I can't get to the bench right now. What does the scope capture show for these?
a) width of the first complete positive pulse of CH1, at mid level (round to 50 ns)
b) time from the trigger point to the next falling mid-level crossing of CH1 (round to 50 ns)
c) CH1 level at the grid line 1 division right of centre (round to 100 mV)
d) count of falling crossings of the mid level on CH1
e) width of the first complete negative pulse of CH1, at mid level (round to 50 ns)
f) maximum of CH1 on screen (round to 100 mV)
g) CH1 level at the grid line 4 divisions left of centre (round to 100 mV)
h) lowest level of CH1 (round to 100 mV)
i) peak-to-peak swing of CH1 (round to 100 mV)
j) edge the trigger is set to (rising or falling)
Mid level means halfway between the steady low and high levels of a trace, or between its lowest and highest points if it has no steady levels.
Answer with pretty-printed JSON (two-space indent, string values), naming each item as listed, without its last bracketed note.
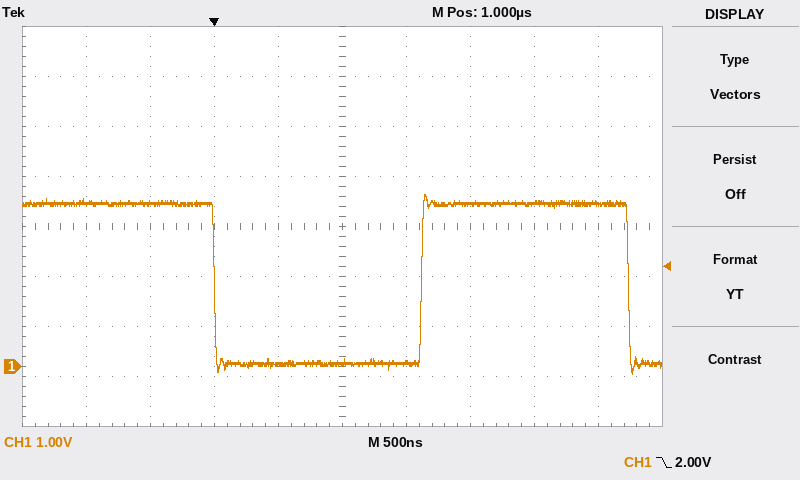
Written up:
{
  "width of the first complete positive pulse of CH1, at mid level": "1.60 µs",
  "time from the trigger point to the next falling mid-level crossing of CH1": "3.25 µs",
  "CH1 level at the grid line 1 division right of centre": "100 mV",
  "count of falling crossings of the mid level on CH1": "2",
  "width of the first complete negative pulse of CH1, at mid level": "1.60 µs",
  "maximum of CH1 on screen": "3.4 V",
  "CH1 level at the grid line 4 divisions left of centre": "3.3 V",
  "lowest level of CH1": "-200 mV",
  "peak-to-peak swing of CH1": "3.6 V",
  "edge the trigger is set to": "falling"
}
